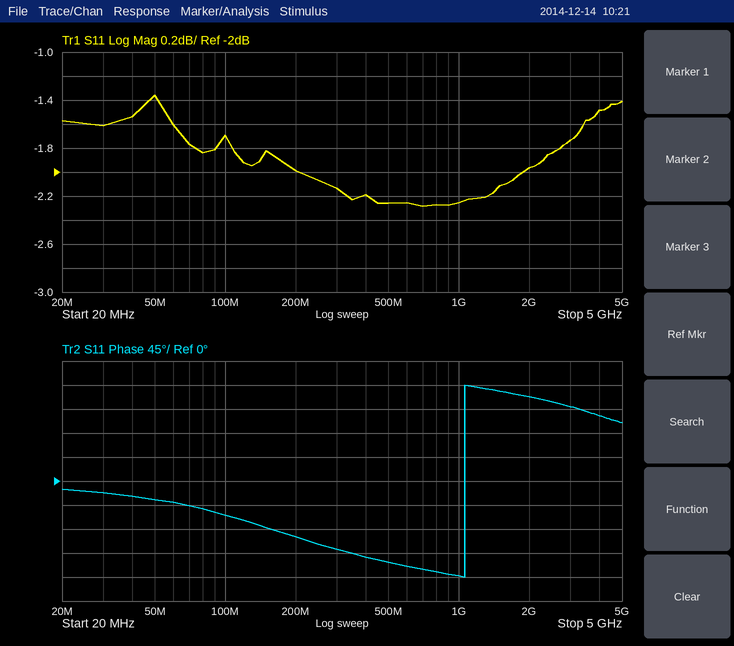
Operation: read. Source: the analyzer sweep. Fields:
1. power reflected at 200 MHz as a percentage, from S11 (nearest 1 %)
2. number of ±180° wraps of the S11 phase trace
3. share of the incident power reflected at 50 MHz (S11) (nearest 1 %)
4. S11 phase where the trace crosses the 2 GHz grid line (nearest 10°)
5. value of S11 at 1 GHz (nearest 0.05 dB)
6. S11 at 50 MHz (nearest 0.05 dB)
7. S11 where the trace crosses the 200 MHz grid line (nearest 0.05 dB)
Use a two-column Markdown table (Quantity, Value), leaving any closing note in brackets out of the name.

| Quantity | Value |
|---|---|
| power reflected at 200 MHz as a percentage, from S11 | 63 % |
| number of ±180° wraps of the S11 phase trace | 1 |
| share of the incident power reflected at 50 MHz (S11) | 73 % |
| S11 phase where the trace crosses the 2 GHz grid line | 160° |
| value of S11 at 1 GHz | -2.25 dB |
| S11 at 50 MHz | -1.35 dB |
| S11 where the trace crosses the 200 MHz grid line | -2.00 dB |
